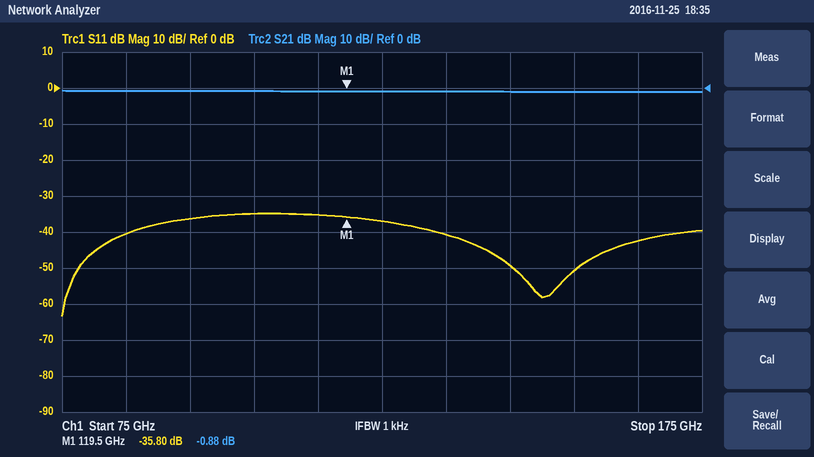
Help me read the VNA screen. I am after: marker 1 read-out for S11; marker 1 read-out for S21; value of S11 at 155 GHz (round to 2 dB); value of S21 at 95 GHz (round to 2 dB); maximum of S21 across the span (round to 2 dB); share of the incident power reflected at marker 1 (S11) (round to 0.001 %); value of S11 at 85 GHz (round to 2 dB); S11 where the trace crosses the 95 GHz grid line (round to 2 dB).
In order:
-35.80 dB
-0.88 dB
-50 dB
0 dB
0 dB
0.026 %
-40 dB
-36 dB
